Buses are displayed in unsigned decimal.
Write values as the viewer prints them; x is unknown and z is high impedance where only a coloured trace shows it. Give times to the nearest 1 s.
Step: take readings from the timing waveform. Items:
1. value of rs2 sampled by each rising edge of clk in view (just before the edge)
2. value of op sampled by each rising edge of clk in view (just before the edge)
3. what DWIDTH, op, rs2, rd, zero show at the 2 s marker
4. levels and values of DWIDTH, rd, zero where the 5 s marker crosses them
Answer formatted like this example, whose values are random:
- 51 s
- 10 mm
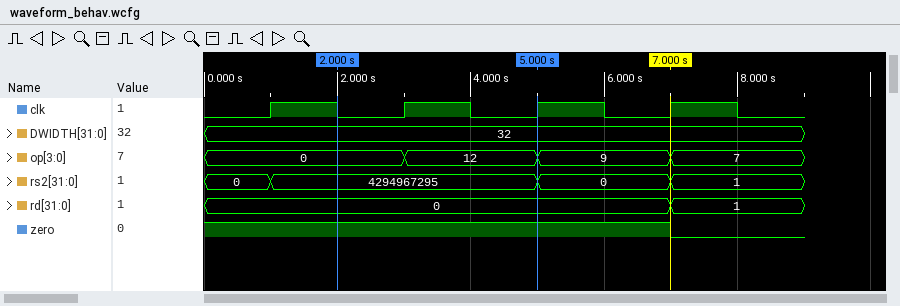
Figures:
- 0, 4294967295, 4294967295, 0
- 0, 0, 12, 9
- DWIDTH=32, op=0, rs2=4294967295, rd=0, zero=1
- DWIDTH=32, rd=0, zero=1
